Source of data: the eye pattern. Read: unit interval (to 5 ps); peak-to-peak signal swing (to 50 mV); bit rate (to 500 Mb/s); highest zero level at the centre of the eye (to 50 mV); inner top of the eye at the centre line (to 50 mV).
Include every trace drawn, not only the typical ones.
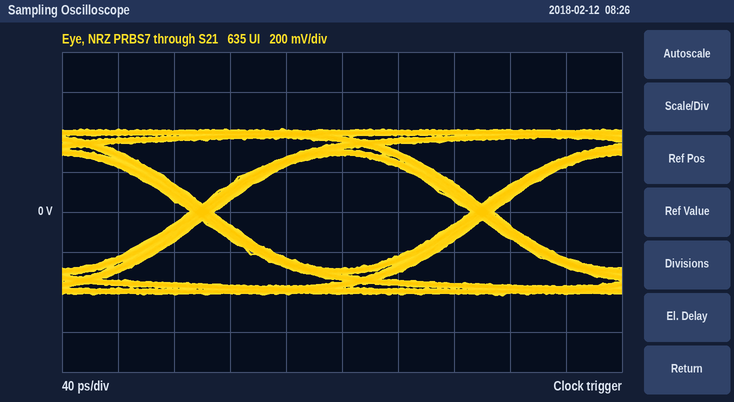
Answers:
200 ps
850 mV
5.0 Gb/s
-300 mV
300 mV
